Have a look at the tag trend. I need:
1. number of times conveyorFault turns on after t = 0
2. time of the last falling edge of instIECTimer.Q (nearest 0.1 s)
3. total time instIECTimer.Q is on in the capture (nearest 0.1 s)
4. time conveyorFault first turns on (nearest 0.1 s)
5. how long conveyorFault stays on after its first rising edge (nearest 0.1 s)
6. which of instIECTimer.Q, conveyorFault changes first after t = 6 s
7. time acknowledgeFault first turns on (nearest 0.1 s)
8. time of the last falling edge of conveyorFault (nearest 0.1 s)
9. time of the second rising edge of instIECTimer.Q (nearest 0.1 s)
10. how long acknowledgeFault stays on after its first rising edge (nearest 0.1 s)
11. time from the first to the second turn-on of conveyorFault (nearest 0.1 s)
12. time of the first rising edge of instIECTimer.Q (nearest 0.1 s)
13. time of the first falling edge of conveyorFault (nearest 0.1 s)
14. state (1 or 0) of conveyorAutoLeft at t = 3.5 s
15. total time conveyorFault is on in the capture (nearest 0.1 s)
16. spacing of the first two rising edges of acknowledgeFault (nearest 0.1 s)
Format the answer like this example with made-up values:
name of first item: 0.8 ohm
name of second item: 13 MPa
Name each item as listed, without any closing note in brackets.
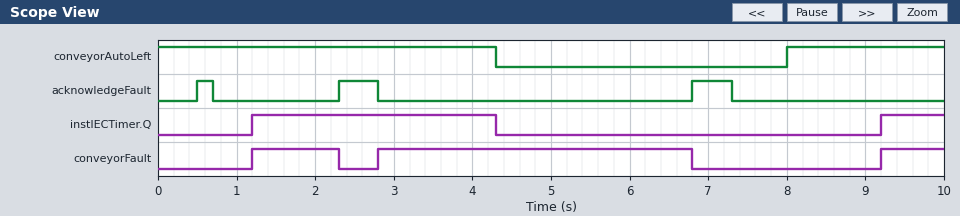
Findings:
number of times conveyorFault turns on after t = 0: 3
time of the last falling edge of instIECTimer.Q: 4.3 s
total time instIECTimer.Q is on in the capture: 3.9 s
time conveyorFault first turns on: 1.2 s
how long conveyorFault stays on after its first rising edge: 1.1 s
which of instIECTimer.Q, conveyorFault changes first after t = 6 s: conveyorFault
time acknowledgeFault first turns on: 0.5 s
time of the last falling edge of conveyorFault: 6.8 s
time of the second rising edge of instIECTimer.Q: 9.2 s
how long acknowledgeFault stays on after its first rising edge: 0.2 s
time from the first to the second turn-on of conveyorFault: 1.6 s
time of the first rising edge of instIECTimer.Q: 1.2 s
time of the first falling edge of conveyorFault: 2.3 s
state (1 or 0) of conveyorAutoLeft at t = 3.5 s: 1
total time conveyorFault is on in the capture: 5.9 s
spacing of the first two rising edges of acknowledgeFault: 1.8 s
